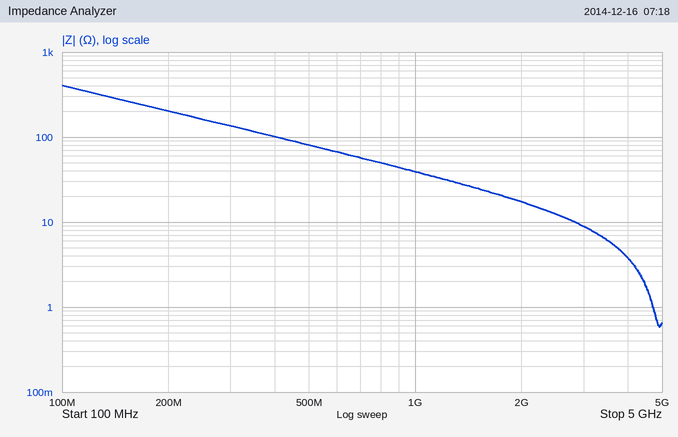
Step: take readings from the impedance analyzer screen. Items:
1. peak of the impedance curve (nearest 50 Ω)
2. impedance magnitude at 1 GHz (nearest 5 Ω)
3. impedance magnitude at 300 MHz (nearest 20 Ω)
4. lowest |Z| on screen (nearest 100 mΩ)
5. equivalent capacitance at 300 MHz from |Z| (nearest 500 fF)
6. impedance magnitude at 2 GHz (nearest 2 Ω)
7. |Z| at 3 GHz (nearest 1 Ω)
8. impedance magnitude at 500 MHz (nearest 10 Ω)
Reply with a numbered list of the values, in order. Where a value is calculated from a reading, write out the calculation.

1. 400 Ω
2. 40 Ω
3. 140 Ω
4. 600 mΩ
5. C = 1/(2π × 300 MHz × 140 Ω) ≈ 3.79 pF, so 4.0 pF to the nearest 500 fF
6. 18 Ω
7. 9 Ω
8. 80 Ω
